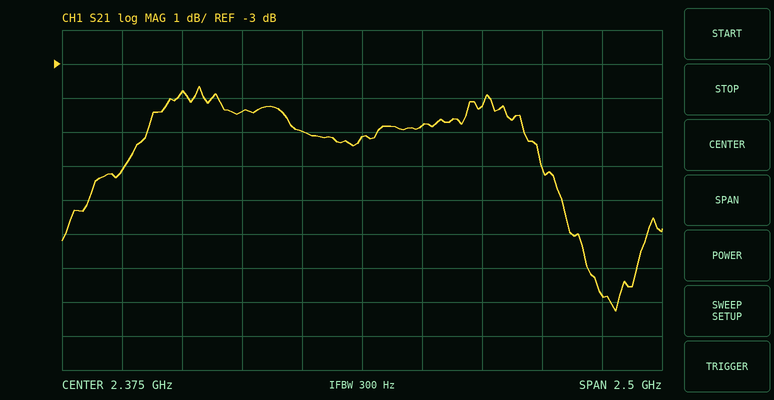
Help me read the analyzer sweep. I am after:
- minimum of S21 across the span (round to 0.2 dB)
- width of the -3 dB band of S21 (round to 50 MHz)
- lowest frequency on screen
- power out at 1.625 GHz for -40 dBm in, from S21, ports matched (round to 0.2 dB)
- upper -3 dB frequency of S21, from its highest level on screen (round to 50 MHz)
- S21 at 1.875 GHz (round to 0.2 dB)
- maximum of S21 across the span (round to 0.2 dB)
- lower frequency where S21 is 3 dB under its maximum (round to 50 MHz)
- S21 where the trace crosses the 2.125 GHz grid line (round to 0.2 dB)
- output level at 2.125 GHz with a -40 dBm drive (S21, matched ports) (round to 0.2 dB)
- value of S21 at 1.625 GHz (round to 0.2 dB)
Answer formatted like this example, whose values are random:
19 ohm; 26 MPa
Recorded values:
-10.2 dB; 1.95 GHz; 1.125 GHz; -43.8 dBm; 3.20 GHz; -4.4 dB; -3.6 dB; 1.25 GHz; -5.0 dB; -45.0 dBm; -3.8 dB
